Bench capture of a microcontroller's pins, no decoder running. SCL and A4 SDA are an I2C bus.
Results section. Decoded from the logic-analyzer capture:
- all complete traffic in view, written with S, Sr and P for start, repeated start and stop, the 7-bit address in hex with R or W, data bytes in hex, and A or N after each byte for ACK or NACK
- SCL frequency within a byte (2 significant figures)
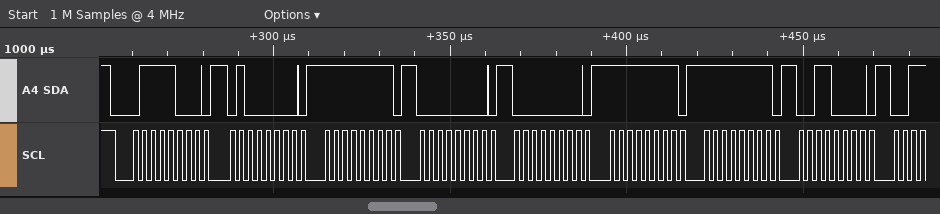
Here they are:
S 3CW A 40 A FF A 00 A 00 A FF A FF A 30 A
400 kHz
